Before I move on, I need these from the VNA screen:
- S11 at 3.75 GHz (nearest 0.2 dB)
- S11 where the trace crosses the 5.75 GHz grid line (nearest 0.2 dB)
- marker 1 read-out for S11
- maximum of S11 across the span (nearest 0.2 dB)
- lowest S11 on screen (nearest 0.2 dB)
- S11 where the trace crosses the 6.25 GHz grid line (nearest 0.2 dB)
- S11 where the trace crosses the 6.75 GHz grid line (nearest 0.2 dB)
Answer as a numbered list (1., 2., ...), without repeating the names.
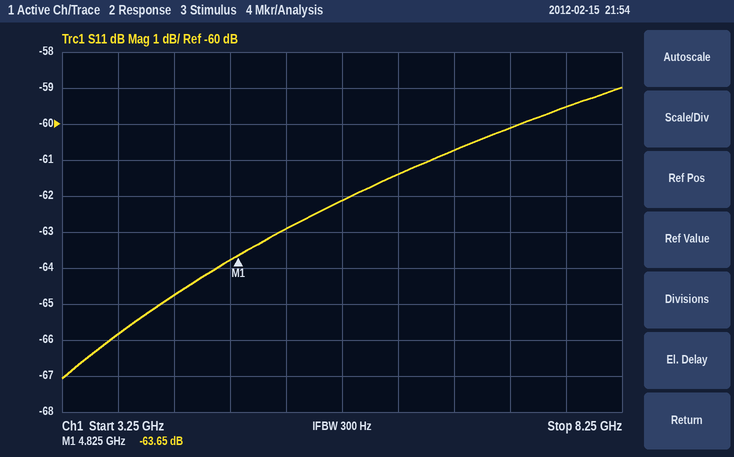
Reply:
1. -65.8 dB
2. -62.2 dB
3. -63.65 dB
4. -59.0 dB
5. -67.0 dB
6. -61.4 dB
7. -60.8 dB
